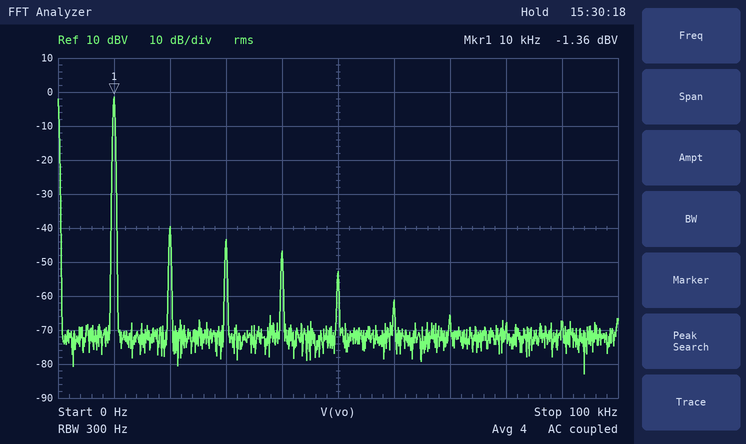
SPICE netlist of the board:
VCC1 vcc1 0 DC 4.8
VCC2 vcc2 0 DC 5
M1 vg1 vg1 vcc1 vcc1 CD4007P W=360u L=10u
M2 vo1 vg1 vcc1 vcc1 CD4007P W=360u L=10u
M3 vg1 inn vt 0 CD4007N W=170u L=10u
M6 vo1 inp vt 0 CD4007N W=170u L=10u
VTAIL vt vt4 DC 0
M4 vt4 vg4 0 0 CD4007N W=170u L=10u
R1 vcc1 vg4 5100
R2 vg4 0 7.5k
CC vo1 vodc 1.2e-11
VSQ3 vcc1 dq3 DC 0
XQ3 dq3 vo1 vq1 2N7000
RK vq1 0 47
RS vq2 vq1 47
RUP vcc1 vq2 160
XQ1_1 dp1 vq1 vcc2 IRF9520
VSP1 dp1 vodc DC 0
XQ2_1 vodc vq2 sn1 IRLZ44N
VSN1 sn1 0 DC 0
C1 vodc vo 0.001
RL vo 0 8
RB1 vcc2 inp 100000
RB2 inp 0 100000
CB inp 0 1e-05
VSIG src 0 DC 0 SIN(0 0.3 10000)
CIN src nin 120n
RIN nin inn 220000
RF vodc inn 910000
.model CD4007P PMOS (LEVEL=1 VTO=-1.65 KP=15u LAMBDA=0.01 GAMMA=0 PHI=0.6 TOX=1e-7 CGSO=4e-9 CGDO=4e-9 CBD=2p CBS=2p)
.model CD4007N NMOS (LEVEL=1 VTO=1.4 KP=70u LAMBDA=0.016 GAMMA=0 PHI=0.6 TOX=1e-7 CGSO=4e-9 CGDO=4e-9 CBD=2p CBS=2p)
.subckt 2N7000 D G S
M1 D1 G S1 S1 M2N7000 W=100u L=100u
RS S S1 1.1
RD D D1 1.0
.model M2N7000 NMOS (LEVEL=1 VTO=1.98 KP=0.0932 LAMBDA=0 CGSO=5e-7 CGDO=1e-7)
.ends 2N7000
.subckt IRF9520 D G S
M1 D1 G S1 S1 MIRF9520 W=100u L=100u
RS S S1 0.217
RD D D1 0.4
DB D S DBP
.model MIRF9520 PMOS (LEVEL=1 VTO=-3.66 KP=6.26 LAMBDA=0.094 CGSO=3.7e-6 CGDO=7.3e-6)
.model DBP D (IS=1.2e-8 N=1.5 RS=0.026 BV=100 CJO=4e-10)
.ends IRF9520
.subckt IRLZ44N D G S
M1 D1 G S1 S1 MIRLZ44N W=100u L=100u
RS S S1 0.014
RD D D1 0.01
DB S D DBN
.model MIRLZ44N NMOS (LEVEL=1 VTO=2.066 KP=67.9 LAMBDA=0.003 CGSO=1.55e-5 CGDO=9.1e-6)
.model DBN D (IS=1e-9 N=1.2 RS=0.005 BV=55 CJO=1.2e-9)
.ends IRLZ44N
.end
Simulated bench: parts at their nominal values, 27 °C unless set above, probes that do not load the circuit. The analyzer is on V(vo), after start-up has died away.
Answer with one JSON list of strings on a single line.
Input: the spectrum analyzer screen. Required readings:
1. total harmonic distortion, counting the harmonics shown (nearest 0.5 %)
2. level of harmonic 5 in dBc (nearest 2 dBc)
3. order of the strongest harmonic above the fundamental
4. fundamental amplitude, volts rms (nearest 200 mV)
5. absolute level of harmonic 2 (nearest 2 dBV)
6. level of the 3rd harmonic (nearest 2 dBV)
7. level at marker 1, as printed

["1.5 %", "-52 dBc", "2", "800 mV", "-40 dBV", "-44 dBV", "-1.36 dBV"]
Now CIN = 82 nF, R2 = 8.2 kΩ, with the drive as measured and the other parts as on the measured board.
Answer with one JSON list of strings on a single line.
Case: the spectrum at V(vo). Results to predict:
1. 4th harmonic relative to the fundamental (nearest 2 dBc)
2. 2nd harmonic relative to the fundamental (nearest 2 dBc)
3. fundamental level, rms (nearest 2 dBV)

["-58 dBc", "-52 dBc", "-2 dBV"]
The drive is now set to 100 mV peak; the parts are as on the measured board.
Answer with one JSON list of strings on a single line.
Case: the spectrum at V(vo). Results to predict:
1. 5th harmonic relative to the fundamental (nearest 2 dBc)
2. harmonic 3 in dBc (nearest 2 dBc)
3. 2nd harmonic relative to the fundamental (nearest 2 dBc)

["-50 dBc", "-40 dBc", "-34 dBc"]
